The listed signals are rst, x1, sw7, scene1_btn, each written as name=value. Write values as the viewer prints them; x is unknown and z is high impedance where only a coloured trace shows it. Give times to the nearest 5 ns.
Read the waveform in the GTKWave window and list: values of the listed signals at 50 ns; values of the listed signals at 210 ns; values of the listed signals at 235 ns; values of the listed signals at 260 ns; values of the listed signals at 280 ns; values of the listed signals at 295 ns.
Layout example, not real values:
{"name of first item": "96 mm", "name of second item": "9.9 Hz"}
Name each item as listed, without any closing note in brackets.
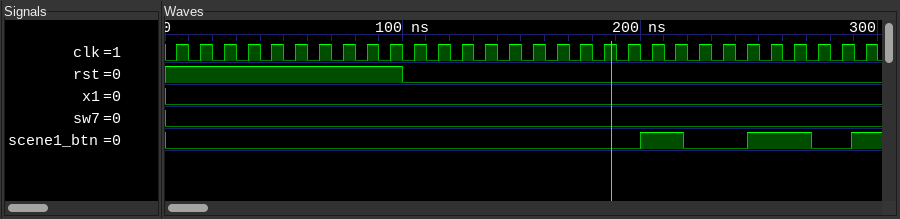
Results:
{"values of the listed signals at 50 ns": "rst=1, x1=0, sw7=0, scene1_btn=0", "values of the listed signals at 210 ns": "rst=0, x1=0, sw7=0, scene1_btn=1", "values of the listed signals at 235 ns": "rst=0, x1=0, sw7=0, scene1_btn=0", "values of the listed signals at 260 ns": "rst=0, x1=0, sw7=0, scene1_btn=1", "values of the listed signals at 280 ns": "rst=0, x1=0, sw7=0, scene1_btn=0", "values of the listed signals at 295 ns": "rst=0, x1=0, sw7=0, scene1_btn=1"}
